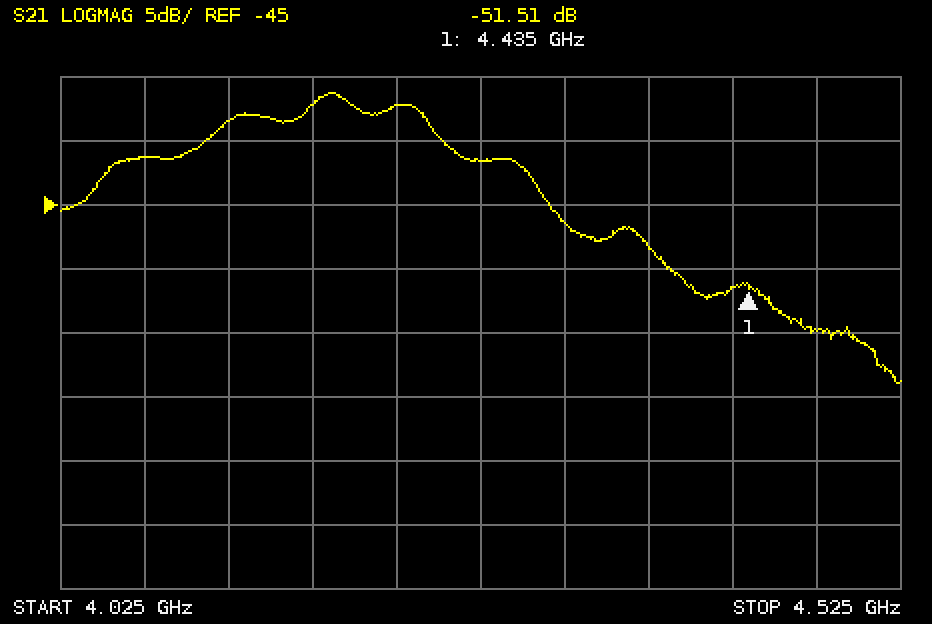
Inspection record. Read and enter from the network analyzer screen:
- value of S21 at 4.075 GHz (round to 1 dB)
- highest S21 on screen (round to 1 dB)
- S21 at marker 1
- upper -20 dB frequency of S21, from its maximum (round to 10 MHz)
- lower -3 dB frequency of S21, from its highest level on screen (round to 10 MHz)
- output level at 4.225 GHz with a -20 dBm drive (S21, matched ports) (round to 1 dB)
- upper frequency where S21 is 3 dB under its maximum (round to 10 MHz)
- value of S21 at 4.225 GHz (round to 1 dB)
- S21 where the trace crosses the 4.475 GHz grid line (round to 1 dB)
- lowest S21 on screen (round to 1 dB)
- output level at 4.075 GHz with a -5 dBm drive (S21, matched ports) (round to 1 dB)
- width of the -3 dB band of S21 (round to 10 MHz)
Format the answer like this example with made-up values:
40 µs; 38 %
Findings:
-41 dB; -36 dB; -51.51 dB; 4.51 GHz; 4.12 GHz; -57 dBm; 4.25 GHz; -37 dB; -55 dB; -59 dB; -46 dBm; 130 MHz
